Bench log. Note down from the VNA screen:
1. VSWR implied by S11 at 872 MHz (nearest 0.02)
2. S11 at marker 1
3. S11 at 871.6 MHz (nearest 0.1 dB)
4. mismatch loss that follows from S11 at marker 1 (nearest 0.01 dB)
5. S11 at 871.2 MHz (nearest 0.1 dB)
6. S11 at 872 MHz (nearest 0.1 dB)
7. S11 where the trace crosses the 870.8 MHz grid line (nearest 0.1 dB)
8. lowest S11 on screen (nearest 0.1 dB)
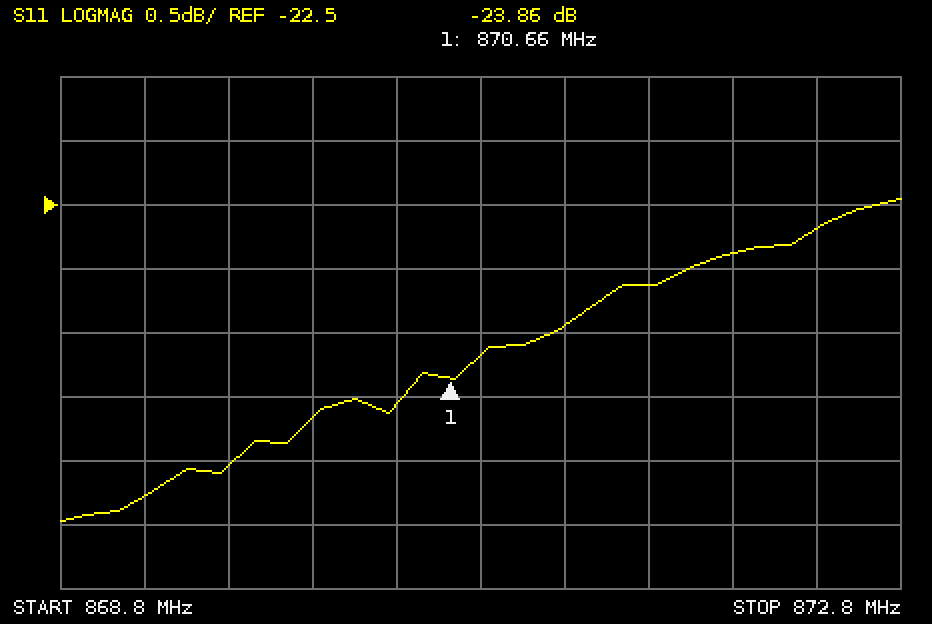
1.16
-23.86 dB
-23.1 dB
0.02 dB
-23.4 dB
-22.9 dB
-23.7 dB
-25.0 dB
